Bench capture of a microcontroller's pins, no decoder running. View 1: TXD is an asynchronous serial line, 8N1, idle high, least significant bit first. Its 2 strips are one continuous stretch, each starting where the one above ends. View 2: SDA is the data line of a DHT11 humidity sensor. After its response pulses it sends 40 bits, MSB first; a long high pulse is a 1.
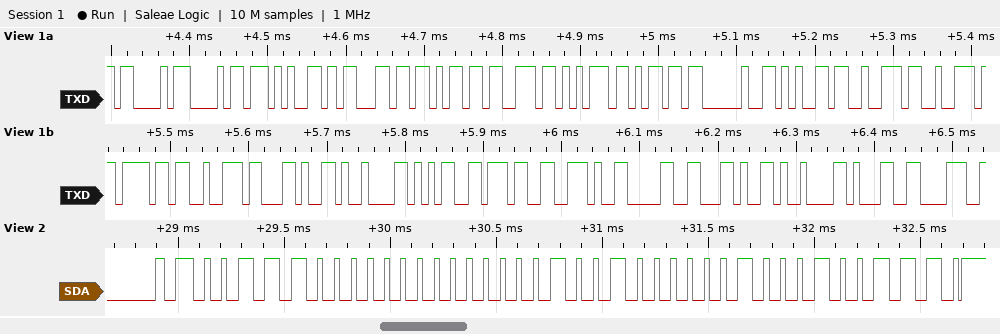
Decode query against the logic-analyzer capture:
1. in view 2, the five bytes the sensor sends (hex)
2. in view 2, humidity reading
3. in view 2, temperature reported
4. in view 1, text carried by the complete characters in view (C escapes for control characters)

38 00 12 04 4E
56 %
18.4 °C
"Checksum error,\t57.0,\t18"
